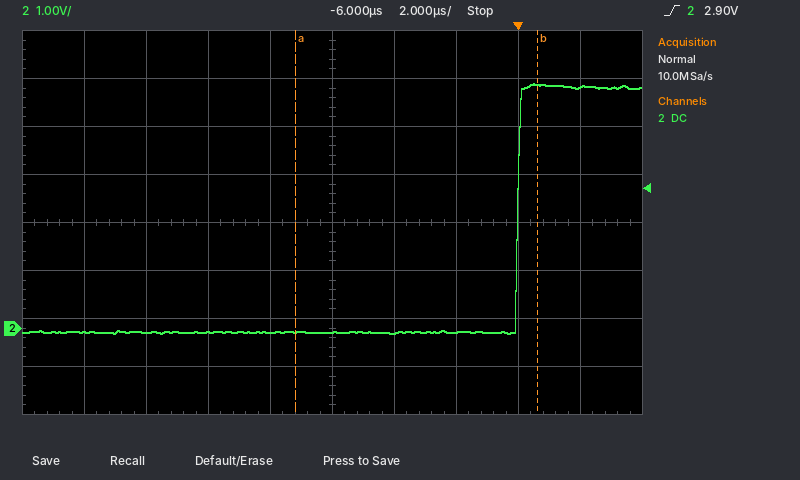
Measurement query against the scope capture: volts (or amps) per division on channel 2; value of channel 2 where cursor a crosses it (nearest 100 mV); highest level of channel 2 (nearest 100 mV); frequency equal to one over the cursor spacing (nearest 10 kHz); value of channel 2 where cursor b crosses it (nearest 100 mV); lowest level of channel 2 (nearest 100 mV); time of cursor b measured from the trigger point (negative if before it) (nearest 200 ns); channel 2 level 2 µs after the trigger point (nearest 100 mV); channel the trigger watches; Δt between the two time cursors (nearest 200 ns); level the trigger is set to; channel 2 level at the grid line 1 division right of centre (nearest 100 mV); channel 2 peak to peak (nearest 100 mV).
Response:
1 V
-100 mV
5.1 V
130 kHz
5.1 V
-100 mV
+600 ns
5.0 V
channel 2
7.8 µs
2.90 V
-100 mV
5.2 V
